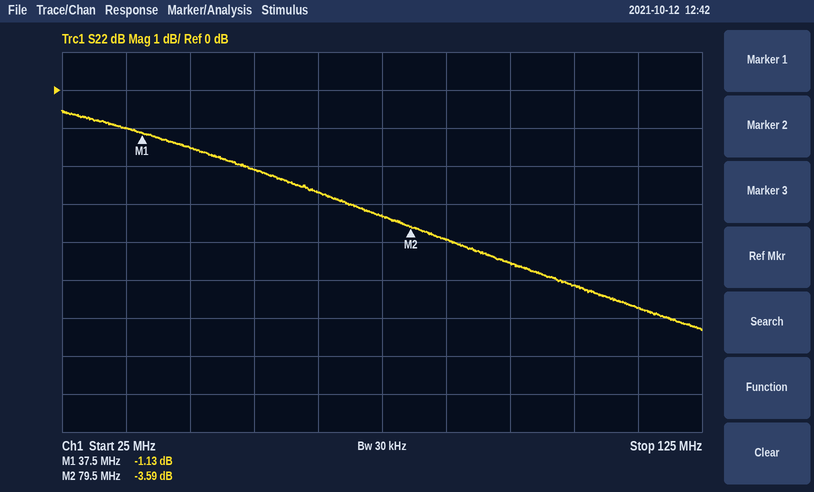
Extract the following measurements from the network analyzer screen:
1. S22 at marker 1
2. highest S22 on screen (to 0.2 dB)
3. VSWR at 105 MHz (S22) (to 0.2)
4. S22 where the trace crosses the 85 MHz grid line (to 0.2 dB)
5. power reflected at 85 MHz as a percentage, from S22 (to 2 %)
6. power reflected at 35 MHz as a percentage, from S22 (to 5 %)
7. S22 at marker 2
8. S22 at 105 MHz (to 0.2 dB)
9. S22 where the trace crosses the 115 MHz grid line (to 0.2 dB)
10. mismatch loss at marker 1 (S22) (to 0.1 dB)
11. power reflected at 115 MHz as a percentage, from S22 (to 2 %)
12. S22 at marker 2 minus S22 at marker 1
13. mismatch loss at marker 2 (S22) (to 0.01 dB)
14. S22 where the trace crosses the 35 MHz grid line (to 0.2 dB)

-1.13 dB
-0.6 dB
3.4
-4.0 dB
40 %
80 %
-3.59 dB
-5.2 dB
-5.8 dB
6.4 dB
26 %
-2.46 dB
2.50 dB
-1.0 dB
